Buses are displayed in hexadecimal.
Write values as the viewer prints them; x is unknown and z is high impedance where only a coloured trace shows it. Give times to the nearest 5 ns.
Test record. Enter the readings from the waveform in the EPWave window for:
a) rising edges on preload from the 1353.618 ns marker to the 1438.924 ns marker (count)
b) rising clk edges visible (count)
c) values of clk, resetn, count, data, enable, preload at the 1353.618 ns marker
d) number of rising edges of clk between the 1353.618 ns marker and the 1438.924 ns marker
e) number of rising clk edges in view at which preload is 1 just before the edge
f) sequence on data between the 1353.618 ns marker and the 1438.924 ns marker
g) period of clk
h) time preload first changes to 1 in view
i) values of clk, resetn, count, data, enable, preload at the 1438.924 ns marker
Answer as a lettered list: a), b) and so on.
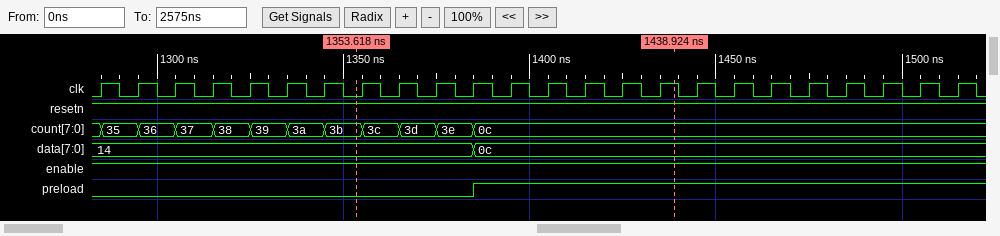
a) 1
b) 24
c) clk=0, resetn=1, count=3b, data=14, enable=1, preload=0
d) 9
e) 13
f) 14, 0c
g) 10 ns
h) 1385 ns
i) clk=1, resetn=1, count=0c, data=0c, enable=1, preload=1
